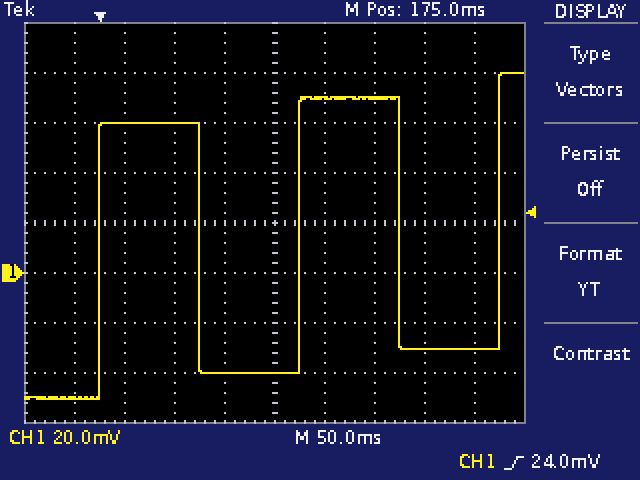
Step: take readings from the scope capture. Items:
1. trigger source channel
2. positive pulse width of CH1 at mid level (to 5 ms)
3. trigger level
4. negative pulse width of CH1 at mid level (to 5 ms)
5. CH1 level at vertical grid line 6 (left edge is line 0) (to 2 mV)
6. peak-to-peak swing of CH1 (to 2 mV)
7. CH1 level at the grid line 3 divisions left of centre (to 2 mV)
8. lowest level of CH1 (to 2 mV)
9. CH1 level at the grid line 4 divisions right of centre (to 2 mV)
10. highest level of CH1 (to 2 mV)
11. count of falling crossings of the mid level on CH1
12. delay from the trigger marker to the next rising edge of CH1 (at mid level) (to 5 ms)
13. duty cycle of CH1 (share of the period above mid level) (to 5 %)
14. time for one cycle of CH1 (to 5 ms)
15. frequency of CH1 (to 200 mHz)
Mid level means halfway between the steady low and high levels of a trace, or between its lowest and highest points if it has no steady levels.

CH1
100 ms
24.0 mV
100 ms
70 mV
130 mV
60 mV
-50 mV
-30 mV
80 mV
2
200 ms
50 %
200 ms
5.0 Hz
